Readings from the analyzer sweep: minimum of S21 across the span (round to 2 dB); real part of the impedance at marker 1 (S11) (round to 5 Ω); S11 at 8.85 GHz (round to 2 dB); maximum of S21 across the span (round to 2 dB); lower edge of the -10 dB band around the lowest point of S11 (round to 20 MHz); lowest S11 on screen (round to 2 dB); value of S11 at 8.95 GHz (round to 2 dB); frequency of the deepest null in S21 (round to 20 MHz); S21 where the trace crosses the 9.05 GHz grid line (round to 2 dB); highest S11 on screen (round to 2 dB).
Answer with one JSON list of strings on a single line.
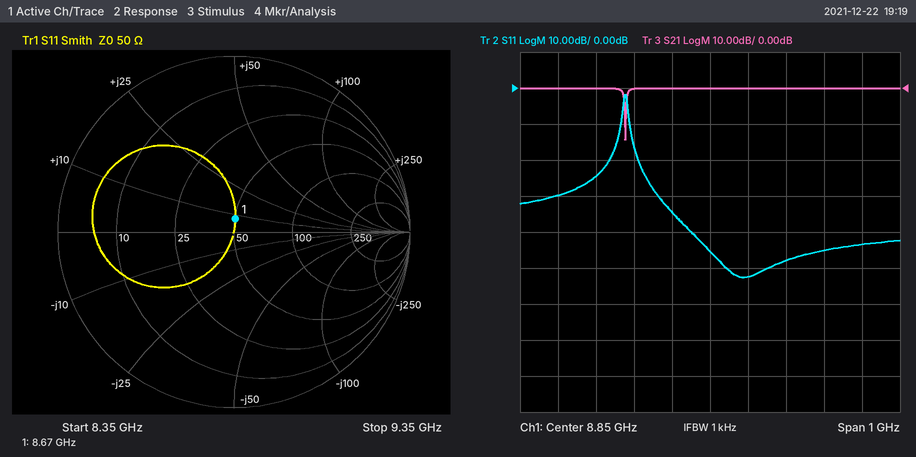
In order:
["-14 dB", "50 Ω", "-46 dB", "0 dB", "8.64 GHz", "-52 dB", "-52 dB", "8.62 GHz", "0 dB", "-2 dB"]
